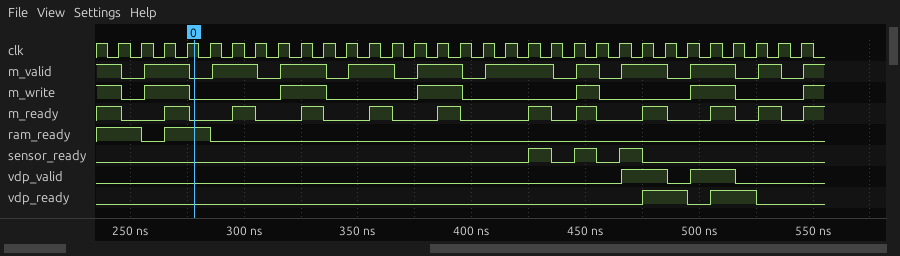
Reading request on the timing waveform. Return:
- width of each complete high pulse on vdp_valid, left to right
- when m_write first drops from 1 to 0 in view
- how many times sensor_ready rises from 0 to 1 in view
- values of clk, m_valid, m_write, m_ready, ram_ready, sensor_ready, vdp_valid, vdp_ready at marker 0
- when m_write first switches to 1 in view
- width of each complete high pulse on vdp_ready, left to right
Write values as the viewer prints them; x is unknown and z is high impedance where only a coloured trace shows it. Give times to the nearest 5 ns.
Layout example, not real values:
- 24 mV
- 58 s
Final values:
- 20 ns, 20 ns
- 245 ns
- 3
- clk=1, m_valid=0, m_write=0, m_ready=0, ram_ready=1, sensor_ready=0, vdp_valid=0, vdp_ready=0
- 255 ns
- 20 ns, 20 ns
